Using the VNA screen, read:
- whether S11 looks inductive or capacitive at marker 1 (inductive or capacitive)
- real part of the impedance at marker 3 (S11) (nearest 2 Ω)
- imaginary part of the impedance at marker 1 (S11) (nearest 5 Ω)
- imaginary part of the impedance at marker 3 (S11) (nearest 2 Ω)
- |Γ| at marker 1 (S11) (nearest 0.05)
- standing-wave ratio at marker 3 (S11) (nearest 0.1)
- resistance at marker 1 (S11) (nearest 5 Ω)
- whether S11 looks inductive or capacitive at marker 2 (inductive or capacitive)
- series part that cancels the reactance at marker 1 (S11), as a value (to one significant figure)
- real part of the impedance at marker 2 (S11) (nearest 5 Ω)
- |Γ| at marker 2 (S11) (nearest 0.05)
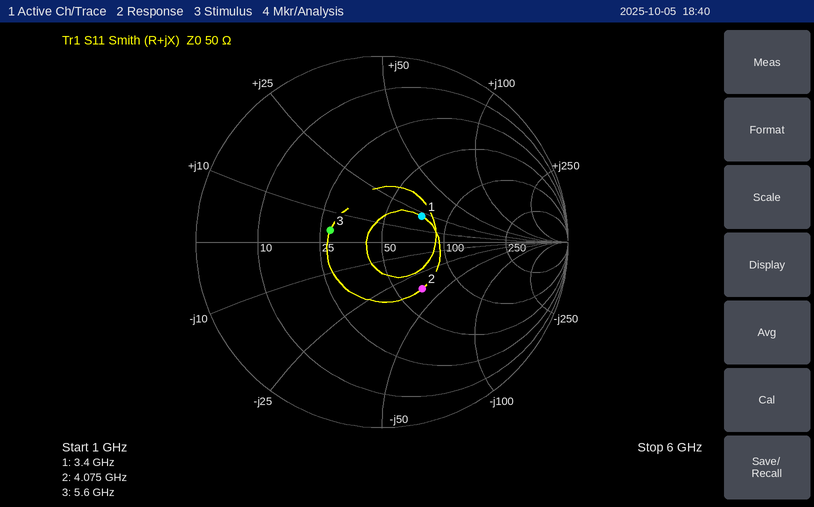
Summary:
inductive
28 Ω
+20 Ω
+4 Ω
0.25
1.8
75 Ω
capacitive
2 pF
65 Ω
0.35
